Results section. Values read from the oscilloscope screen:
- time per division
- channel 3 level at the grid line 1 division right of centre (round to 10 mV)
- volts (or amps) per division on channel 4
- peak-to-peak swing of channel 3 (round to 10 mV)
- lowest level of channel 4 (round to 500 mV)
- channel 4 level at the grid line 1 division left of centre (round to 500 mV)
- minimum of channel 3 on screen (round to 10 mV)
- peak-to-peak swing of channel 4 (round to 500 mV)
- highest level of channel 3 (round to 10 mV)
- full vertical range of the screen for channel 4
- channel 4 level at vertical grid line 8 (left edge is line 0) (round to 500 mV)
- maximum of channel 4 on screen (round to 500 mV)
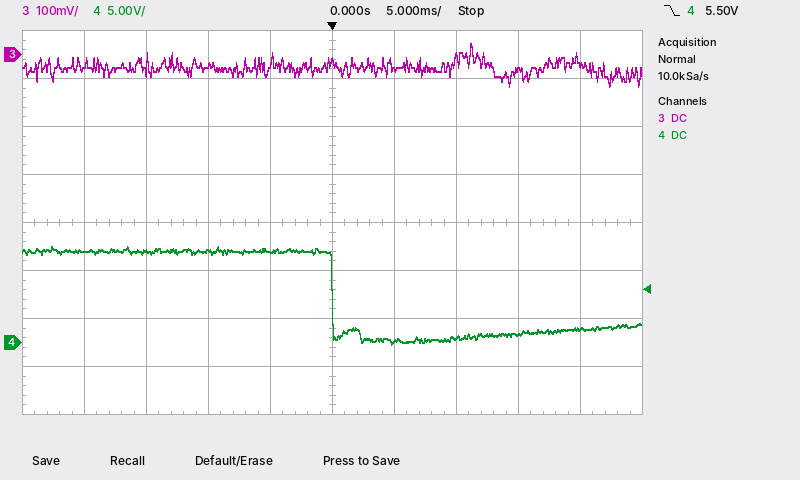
5 ms
-30 mV
5 V
90 mV
0.0 V
9.5 V
-70 mV
10.0 V
20 mV
40 V
1.0 V
10.0 V
